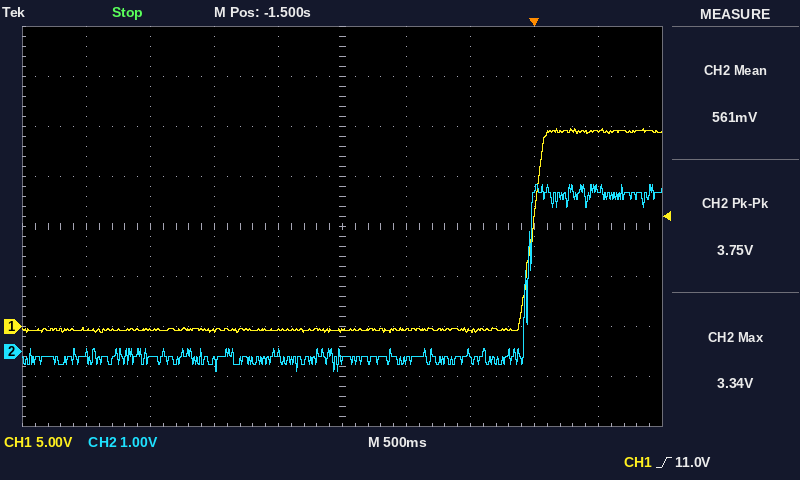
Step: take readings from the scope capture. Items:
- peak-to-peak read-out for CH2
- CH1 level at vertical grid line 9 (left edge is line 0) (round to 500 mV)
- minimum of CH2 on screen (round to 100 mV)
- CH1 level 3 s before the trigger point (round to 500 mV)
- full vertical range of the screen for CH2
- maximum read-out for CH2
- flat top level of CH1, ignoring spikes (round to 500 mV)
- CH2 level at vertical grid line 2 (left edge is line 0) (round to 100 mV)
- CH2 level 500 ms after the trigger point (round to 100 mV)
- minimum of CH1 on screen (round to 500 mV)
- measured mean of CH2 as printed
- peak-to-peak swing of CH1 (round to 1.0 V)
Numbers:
3.75 V
19.5 V
-400 mV
-500 mV
8 V
3.34 V
19.5 V
-200 mV
3.3 V
-500 mV
561 mV
20.0 V
